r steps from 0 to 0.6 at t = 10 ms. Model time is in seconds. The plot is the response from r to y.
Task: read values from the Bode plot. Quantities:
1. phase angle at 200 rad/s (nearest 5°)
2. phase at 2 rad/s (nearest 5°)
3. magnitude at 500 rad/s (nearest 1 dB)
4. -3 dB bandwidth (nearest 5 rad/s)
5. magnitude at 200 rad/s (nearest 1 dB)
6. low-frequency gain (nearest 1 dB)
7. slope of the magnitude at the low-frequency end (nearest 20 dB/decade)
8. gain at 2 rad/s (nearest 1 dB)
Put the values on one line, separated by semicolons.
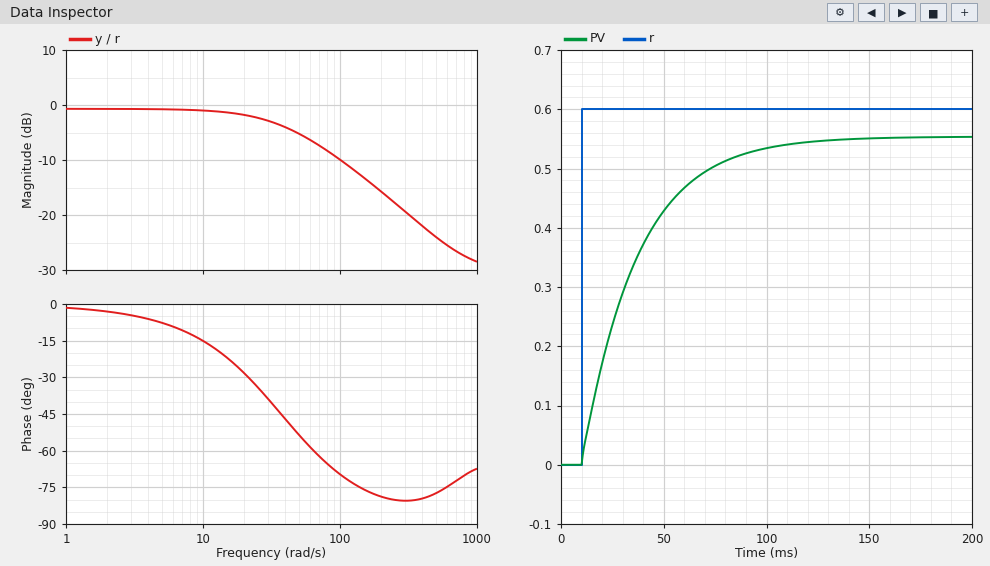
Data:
-80°; -5°; -24 dB; 35 rad/s; -16 dB; -1 dB; 0 dB/decade; -1 dB
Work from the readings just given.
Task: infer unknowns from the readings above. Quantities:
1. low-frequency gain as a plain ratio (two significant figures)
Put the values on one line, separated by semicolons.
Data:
0.89
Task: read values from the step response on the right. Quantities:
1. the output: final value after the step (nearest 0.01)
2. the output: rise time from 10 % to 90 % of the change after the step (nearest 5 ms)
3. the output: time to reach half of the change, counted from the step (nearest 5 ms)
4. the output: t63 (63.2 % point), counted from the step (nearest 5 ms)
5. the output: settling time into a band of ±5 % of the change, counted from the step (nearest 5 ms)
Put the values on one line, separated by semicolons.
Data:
0.55; 60 ms; 20 ms; 25 ms; 80 ms
